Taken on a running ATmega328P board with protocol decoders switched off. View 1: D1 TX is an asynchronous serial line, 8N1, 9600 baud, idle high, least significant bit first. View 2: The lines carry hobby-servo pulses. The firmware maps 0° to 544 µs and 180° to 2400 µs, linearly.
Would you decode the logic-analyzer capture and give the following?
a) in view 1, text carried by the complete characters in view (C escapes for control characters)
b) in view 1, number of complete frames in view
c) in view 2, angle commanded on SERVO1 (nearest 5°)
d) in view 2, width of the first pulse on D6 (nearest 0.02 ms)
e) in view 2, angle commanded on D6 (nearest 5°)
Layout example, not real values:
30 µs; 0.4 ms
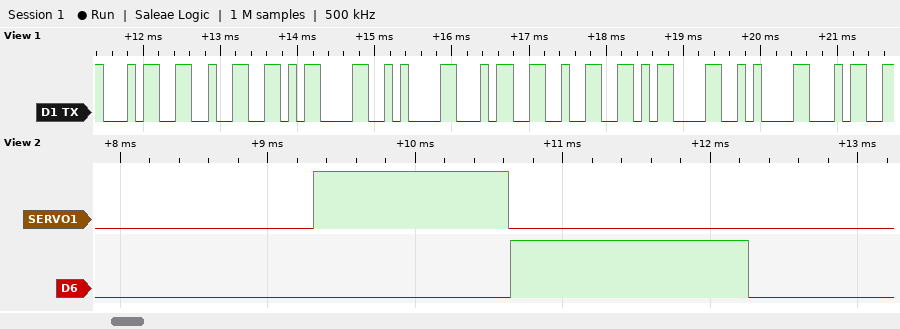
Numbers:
"42\r\n42\r\n4"; 9; 75°; 1.62 ms; 105°
